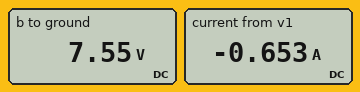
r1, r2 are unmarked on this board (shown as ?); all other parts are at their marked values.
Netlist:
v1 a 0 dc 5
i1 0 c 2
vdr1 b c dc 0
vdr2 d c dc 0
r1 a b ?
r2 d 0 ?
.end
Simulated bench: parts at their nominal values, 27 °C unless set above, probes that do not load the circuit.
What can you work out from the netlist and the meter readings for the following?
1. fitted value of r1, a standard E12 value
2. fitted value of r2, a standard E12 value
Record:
3.9 Ω
5.6 Ω
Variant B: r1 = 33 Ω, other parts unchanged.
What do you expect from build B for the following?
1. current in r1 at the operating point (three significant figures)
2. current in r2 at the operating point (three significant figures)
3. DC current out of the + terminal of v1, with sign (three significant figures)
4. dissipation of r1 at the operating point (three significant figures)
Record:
161 mA
1.84 A
-161 mA
851 mW
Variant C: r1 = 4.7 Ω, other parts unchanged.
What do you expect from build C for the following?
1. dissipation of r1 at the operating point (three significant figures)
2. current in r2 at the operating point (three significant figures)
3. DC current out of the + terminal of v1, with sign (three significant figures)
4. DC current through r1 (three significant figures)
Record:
1.70 W
1.40 A
-602 mA
602 mA
